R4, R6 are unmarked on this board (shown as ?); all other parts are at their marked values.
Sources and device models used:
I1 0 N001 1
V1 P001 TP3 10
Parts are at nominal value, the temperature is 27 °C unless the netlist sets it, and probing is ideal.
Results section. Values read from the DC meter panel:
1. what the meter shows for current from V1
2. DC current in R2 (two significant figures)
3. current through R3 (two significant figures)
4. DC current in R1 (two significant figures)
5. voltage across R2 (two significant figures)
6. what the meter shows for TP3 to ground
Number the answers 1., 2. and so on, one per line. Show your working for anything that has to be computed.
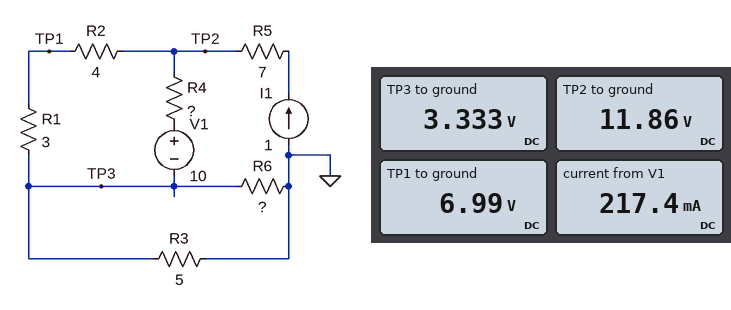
1. 217.4 mA
2. (11.86 V - 6.99 V) / 4 Ω = 1.2 A
3. (3.333 V) / 5 Ω = 670 mA
4. (6.99 V - 3.333 V) / 3 Ω = 1.2 A
5. 11.86 V - 6.99 V = 4.9 V
6. 3.333 V
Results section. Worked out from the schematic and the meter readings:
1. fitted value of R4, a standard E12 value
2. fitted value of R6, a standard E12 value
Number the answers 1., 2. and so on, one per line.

1. 6.8 Ω
2. 10 Ω
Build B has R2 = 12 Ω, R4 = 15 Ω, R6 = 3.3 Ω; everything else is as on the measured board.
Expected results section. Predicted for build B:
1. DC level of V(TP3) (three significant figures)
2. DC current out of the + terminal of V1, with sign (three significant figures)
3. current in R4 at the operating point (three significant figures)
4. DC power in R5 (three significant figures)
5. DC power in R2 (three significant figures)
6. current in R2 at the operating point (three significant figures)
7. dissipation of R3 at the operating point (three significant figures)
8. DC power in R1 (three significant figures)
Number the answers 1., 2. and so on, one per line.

1. 1.99 V
2. -167 mA
3. 167 mA
4. 7.00 W
5. 8.33 W
6. 833 mA
7. 790 mW
8. 2.08 W
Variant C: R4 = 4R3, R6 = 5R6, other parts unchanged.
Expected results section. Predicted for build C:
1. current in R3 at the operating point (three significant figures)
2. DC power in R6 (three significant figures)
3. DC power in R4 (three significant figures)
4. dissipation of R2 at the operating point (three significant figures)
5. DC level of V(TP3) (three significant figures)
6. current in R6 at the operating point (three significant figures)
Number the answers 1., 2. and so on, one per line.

1. 528 mA
2. 1.25 W
3. 303 mW
4. 6.41 W
5. 2.64 V
6. 472 mA
